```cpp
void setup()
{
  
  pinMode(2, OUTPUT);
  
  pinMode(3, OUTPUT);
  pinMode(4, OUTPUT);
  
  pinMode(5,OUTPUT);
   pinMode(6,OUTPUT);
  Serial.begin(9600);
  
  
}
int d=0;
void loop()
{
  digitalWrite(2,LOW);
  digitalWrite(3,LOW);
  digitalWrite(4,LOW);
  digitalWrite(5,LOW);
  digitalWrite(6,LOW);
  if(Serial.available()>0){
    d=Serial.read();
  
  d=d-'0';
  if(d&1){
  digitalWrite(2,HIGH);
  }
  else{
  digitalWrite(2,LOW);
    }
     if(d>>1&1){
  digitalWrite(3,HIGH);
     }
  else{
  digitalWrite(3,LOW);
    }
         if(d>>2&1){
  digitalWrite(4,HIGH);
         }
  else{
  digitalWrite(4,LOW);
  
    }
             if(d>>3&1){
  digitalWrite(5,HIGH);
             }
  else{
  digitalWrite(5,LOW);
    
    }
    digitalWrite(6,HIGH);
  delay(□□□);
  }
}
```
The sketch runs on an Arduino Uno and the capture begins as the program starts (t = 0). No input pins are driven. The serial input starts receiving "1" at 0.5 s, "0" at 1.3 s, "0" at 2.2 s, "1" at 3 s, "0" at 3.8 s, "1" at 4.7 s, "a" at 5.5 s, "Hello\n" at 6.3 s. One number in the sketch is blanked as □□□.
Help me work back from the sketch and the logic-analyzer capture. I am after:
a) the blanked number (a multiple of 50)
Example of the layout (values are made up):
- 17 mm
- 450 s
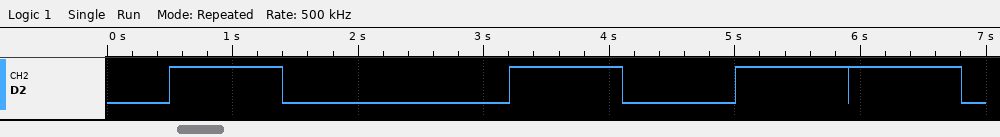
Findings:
- 900
